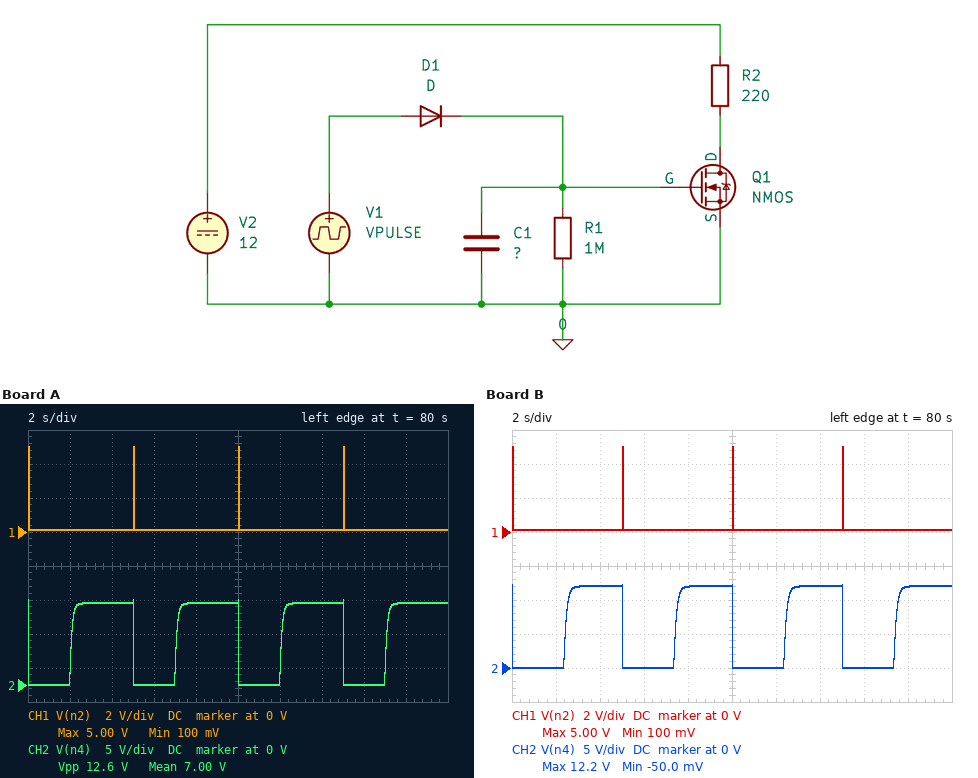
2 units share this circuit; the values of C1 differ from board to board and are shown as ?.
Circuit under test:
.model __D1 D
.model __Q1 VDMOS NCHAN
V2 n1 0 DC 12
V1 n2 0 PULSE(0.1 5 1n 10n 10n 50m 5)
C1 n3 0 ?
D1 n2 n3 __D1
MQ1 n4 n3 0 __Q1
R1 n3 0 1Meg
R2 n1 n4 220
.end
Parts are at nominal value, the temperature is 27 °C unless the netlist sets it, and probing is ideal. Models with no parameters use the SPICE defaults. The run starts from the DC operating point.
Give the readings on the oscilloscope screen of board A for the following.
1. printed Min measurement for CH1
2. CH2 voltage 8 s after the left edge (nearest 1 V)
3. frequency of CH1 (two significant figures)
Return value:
100 mV
12 V
200 mHz
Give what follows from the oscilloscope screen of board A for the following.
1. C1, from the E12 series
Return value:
4.7 µF
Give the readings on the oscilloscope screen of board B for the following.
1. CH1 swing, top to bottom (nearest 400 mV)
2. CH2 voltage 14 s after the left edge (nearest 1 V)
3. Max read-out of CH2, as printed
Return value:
4.8 V
12 V
12.2 V
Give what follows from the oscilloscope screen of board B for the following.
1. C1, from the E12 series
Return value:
5.6 µF
